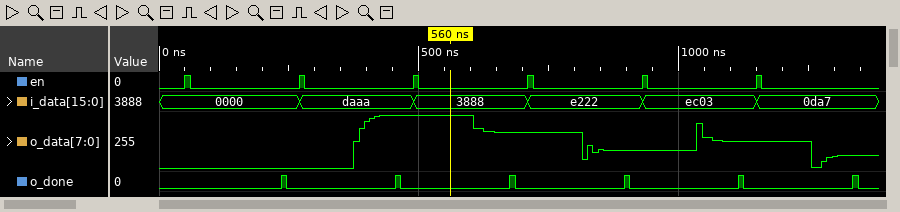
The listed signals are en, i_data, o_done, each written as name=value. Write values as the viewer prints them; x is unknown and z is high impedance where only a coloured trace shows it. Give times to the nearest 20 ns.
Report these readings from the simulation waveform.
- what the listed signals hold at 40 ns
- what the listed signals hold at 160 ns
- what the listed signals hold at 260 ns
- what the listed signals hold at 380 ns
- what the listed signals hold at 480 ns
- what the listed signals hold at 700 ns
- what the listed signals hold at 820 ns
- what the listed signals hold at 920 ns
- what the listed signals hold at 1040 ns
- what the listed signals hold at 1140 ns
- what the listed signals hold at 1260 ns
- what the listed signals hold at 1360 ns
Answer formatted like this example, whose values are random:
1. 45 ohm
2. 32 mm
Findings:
1. en=0, i_data=0000, o_done=0
2. en=0, i_data=0000, o_done=0
3. en=0, i_data=0000, o_done=0
4. en=0, i_data=daaa, o_done=0
5. en=0, i_data=daaa, o_done=0
6. en=0, i_data=3888, o_done=0
7. en=0, i_data=e222, o_done=0
8. en=0, i_data=e222, o_done=0
9. en=0, i_data=ec03, o_done=0
10. en=0, i_data=ec03, o_done=0
11. en=0, i_data=0da7, o_done=0
12. en=0, i_data=0da7, o_done=0
